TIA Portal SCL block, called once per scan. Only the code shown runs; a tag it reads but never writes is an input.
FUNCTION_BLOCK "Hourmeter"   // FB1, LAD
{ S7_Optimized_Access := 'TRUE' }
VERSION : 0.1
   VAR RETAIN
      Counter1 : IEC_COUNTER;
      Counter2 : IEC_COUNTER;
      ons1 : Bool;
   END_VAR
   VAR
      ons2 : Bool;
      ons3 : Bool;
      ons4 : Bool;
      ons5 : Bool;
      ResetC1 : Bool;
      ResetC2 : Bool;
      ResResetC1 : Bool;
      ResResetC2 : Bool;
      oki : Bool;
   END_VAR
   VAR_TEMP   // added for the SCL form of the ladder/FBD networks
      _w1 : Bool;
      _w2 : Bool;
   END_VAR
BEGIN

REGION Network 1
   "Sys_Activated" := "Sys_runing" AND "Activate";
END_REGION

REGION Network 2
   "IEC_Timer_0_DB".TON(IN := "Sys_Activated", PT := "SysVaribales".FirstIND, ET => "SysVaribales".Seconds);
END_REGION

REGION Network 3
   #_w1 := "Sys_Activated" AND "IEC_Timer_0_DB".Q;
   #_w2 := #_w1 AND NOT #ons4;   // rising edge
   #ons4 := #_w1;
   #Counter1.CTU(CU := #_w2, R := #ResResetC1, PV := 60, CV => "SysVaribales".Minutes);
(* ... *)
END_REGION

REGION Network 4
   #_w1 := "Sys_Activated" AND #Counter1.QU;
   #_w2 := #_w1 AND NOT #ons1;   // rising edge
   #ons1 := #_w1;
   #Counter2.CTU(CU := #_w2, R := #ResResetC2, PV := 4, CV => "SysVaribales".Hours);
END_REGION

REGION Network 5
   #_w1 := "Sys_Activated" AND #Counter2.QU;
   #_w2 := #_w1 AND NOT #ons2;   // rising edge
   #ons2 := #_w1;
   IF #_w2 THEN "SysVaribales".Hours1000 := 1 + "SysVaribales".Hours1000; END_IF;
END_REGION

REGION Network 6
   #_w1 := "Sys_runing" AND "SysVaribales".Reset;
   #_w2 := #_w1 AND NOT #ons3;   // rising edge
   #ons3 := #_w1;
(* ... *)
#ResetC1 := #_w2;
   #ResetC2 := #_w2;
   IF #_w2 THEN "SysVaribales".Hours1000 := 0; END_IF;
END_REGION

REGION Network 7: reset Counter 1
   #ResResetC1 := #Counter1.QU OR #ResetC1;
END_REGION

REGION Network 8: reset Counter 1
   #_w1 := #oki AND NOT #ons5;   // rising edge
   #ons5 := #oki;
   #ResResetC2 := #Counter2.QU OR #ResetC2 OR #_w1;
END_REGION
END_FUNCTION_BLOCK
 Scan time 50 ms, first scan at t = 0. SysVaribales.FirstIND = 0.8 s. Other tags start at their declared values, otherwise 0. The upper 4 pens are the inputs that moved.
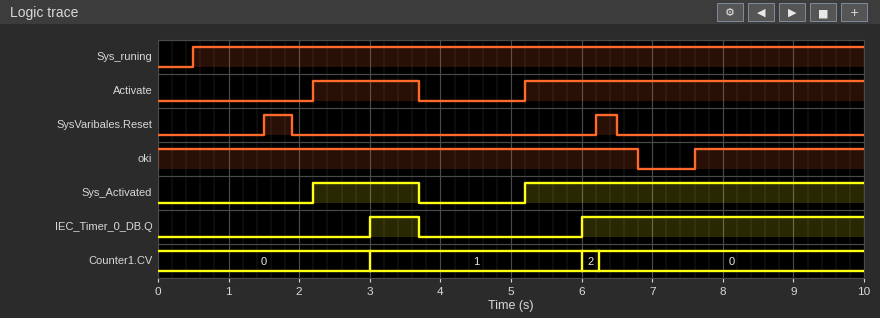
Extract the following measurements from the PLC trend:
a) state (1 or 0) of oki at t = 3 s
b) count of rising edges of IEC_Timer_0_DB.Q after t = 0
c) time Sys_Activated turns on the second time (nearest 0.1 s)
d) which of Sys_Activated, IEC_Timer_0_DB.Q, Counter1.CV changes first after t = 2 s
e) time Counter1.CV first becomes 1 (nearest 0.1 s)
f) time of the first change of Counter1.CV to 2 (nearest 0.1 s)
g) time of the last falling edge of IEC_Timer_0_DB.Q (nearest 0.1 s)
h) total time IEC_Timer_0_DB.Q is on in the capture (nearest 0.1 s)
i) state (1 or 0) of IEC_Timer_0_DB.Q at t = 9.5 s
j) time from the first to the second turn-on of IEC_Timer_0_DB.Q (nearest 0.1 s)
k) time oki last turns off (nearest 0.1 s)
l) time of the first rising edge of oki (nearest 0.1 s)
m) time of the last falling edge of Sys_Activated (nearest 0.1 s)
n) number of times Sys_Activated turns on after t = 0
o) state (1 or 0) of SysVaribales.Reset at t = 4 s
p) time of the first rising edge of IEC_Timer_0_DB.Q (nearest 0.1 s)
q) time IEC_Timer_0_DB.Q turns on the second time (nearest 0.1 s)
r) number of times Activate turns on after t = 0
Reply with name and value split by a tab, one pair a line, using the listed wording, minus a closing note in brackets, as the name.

state (1 or 0) of oki at t = 3 s	1
count of rising edges of IEC_Timer_0_DB.Q after t = 0	2
time Sys_Activated turns on the second time	5.2 s
which of Sys_Activated, IEC_Timer_0_DB.Q, Counter1.CV changes first after t = 2 s	Sys_Activated
time Counter1.CV first becomes 1	3.0 s
time of the first change of Counter1.CV to 2	6.0 s
time of the last falling edge of IEC_Timer_0_DB.Q	3.7 s
total time IEC_Timer_0_DB.Q is on in the capture	4.7 s
state (1 or 0) of IEC_Timer_0_DB.Q at t = 9.5 s	1
time from the first to the second turn-on of IEC_Timer_0_DB.Q	3.0 s
time oki last turns off	6.8 s
time of the first rising edge of oki	7.6 s
time of the last falling edge of Sys_Activated	3.7 s
number of times Sys_Activated turns on after t = 0	2
state (1 or 0) of SysVaribales.Reset at t = 4 s	0
time of the first rising edge of IEC_Timer_0_DB.Q	3.0 s
time IEC_Timer_0_DB.Q turns on the second time	6.0 s
number of times Activate turns on after t = 0	2
